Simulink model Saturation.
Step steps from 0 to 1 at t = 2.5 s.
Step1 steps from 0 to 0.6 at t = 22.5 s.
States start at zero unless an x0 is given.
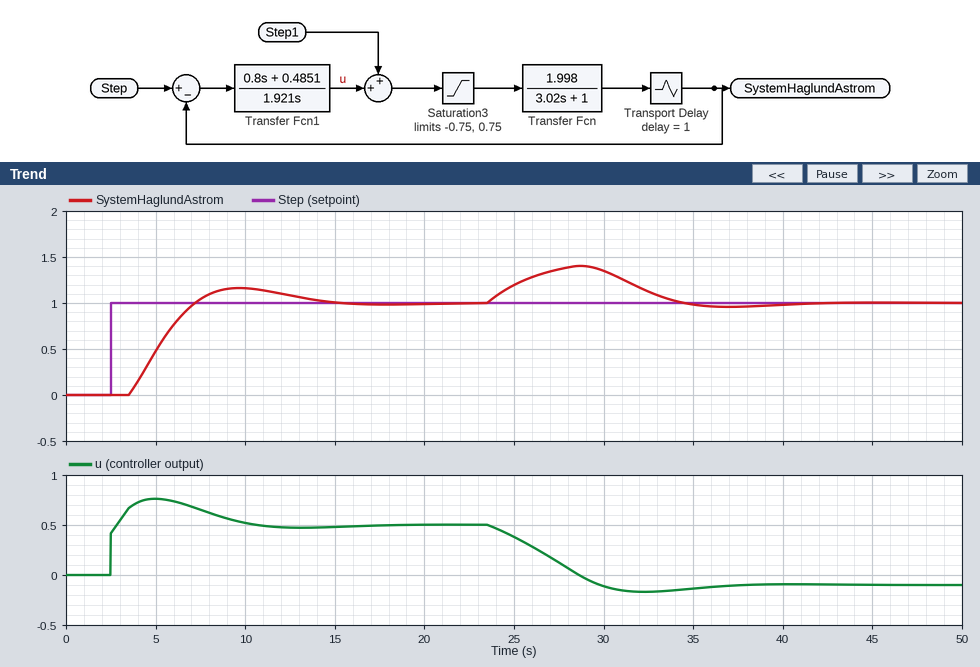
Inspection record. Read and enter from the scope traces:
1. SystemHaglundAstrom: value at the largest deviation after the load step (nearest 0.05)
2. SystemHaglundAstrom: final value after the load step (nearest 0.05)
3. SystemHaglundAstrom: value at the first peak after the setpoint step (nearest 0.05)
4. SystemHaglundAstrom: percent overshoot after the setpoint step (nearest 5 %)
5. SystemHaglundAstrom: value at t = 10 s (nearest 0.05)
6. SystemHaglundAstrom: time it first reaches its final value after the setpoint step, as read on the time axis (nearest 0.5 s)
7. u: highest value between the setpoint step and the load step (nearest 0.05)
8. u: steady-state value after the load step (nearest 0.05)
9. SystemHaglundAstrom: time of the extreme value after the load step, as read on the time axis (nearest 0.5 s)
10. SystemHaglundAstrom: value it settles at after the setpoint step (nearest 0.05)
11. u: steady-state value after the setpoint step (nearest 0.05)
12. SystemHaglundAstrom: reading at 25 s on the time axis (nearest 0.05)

1.40
1.00
1.15
15 %
1.15
7.0 s
0.75
-0.10
28.5 s
1.00
0.50
1.20
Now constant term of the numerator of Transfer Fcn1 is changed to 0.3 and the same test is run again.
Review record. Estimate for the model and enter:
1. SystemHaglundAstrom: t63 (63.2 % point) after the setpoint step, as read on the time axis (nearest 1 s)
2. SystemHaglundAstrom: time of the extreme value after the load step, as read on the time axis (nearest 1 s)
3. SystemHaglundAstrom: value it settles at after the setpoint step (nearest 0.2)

6 s
30 s
1.0
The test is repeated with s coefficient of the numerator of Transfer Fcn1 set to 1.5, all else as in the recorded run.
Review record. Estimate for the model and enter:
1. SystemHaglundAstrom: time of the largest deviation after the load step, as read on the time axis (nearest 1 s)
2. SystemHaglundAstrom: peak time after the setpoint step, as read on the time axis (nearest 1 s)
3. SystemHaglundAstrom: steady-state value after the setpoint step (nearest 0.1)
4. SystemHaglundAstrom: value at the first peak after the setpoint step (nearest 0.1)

28 s
8 s
1.0
1.1
